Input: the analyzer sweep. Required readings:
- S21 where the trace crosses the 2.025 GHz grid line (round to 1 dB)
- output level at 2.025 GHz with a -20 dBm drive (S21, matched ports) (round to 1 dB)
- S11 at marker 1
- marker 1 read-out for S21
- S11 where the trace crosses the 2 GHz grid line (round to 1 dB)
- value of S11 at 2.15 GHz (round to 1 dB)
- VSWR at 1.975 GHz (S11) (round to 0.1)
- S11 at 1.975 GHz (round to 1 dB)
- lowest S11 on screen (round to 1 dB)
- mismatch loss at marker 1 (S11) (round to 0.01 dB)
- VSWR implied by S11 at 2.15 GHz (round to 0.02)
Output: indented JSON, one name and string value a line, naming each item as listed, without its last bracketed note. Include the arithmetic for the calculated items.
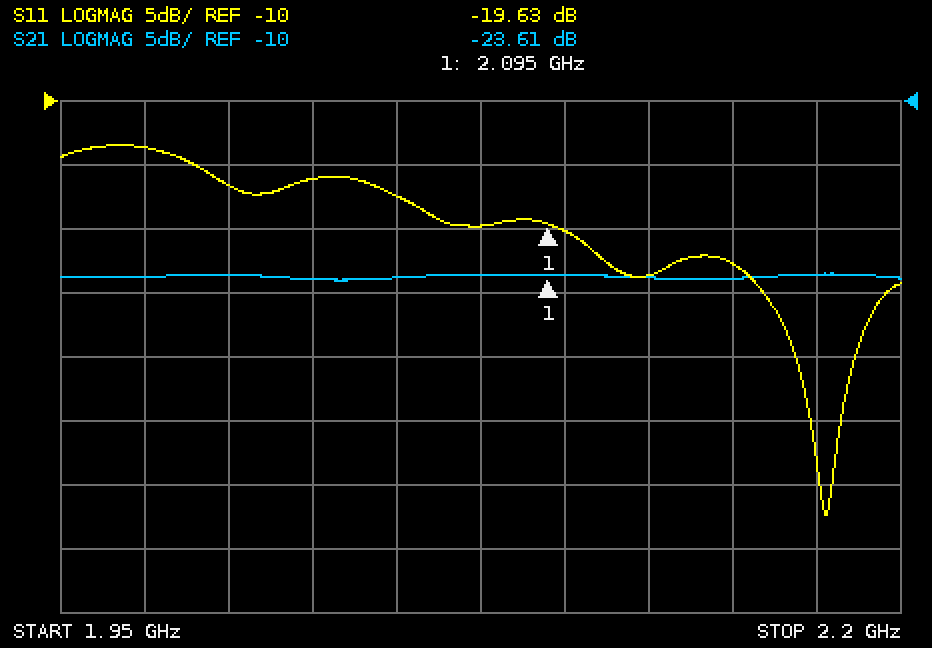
{
  "S21 where the trace crosses the 2.025 GHz grid line": "-24 dB",
  "output level at 2.025 GHz with a -20 dBm drive (S21, matched ports)": "-20 dBm + (-24 dB) = -44 dBm",
  "S11 at marker 1": "-19.63 dB",
  "marker 1 read-out for S21": "-23.61 dB",
  "S11 where the trace crosses the 2 GHz grid line": "-17 dB",
  "value of S11 at 2.15 GHz": "-23 dB",
  "VSWR at 1.975 GHz (S11)": "|Γ| = 10^(-14/20) = 0.1995; VSWR = (1 + 0.1995)/(1 − 0.1995) ≈ 1.5",
  "S11 at 1.975 GHz": "-14 dB",
  "lowest S11 on screen": "-42 dB",
  "mismatch loss at marker 1 (S11)": "−10 log10(1 − 10^(-19.63/10)) ≈ 0.05 dB",
  "VSWR implied by S11 at 2.15 GHz": "|Γ| = 10^(-23/20) = 0.0708; VSWR = (1 + 0.0708)/(1 − 0.0708) ≈ 1.15, so 1.16 to the nearest 0.02"
}
